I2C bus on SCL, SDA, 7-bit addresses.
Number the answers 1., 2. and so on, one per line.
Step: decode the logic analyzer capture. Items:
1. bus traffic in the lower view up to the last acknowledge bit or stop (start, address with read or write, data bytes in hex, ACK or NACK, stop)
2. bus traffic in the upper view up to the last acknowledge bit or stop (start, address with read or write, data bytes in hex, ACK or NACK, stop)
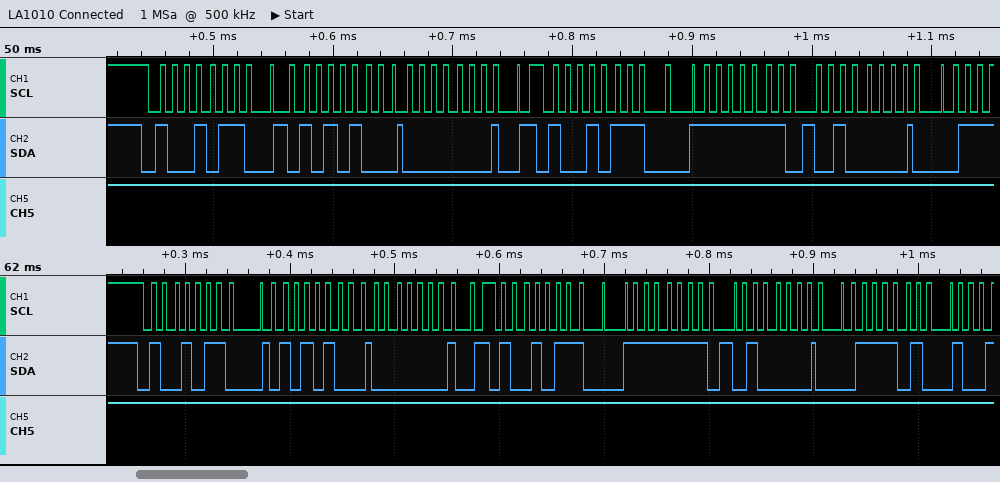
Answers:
1. start, address 4B write ACK, 54 ACK, 01 ACK, repeated start, address 4B read ACK, FF ACK, 20 ACK, 3D ACK
2. start, address 4B write ACK, 54 ACK, 01 ACK, repeated start, address 4B read ACK, FF ACK, 20 ACK
